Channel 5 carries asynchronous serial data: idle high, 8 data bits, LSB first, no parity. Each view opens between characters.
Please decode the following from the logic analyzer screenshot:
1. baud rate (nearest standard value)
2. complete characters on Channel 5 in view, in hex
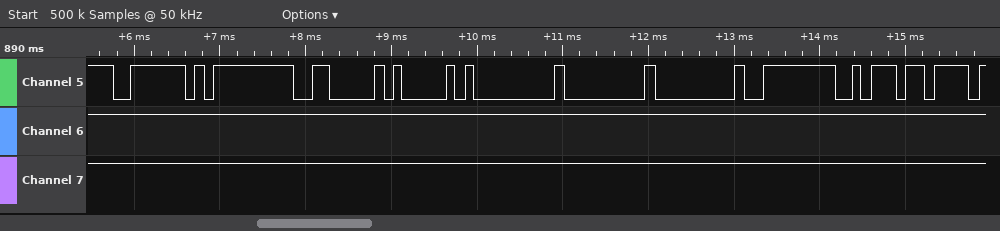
9600 baud
7E, FF, 06, 41, 00, 00, 00, FE, BA
